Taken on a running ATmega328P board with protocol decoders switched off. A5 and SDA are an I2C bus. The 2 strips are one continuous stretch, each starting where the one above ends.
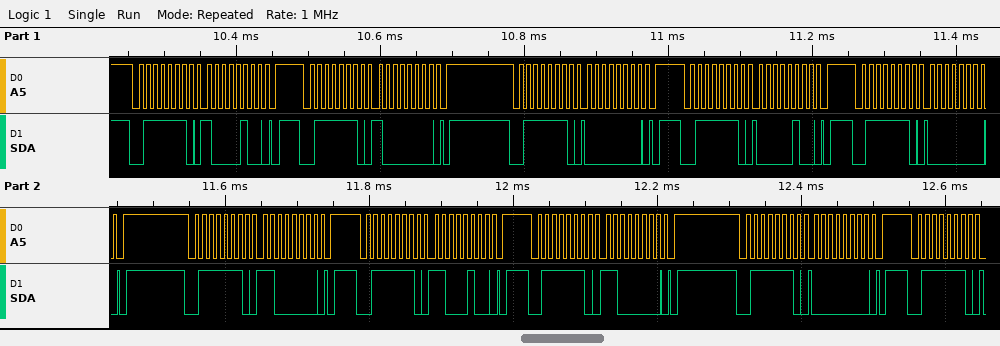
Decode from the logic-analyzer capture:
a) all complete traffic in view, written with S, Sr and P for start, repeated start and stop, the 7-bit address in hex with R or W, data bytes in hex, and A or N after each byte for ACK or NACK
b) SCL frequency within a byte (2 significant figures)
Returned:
S 3FW A 84 A P S 3FW A 80 A P S 3FW A 00 A P S 3FW A 04 A P S 3FW A 00 A P S 3FW A C0 A P S 3FW A C4 A P S 3FW A C0 A P S 3FW A 00 A P S 3FW A
100 kHz
